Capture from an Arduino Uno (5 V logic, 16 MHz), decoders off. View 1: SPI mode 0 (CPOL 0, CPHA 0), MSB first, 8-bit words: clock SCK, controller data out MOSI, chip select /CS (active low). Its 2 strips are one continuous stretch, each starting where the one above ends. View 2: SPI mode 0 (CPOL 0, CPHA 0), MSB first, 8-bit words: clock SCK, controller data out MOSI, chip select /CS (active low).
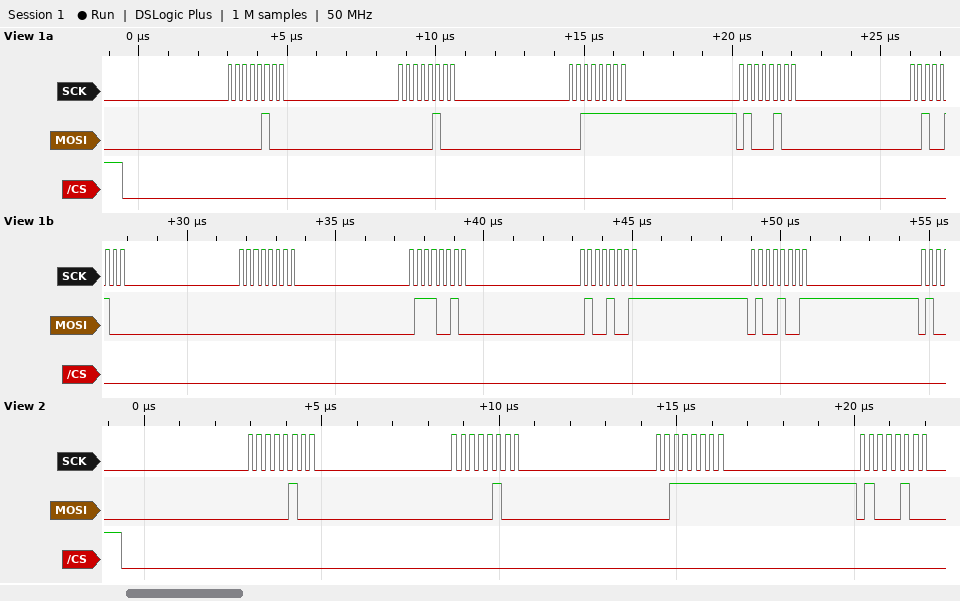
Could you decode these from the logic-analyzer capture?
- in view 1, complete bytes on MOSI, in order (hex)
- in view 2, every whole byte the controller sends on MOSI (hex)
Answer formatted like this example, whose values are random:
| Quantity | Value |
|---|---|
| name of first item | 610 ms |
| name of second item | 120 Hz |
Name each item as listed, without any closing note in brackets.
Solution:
| Quantity | Value |
|---|---|
| in view 1, complete bytes on MOSI, in order | 04 04 3F 44 24 00 72 49 49 |
| in view 2, every whole byte the controller sends on MOSI | 04 04 3F 44 |
